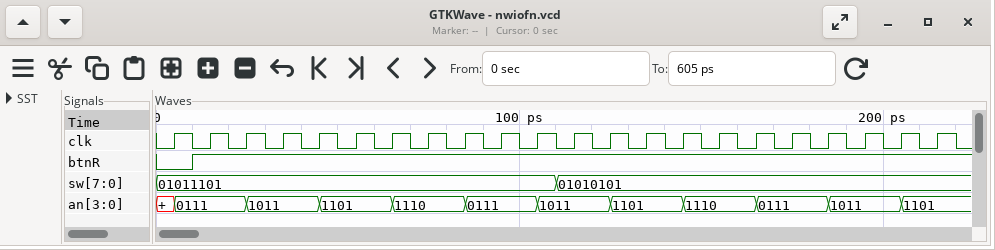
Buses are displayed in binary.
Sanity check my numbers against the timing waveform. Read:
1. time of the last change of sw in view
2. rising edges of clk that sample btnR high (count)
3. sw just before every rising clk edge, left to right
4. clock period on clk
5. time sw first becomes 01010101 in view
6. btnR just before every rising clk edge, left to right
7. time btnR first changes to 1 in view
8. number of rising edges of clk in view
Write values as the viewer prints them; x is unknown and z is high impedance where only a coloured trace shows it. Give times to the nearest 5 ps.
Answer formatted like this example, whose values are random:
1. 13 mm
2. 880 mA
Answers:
1. 110 ps
2. 21
3. 01011101, 01011101, 01011101, 01011101, 01011101, 01011101, 01011101, 01011101, 01011101, 01011101, 01011101, 01010101, 01010101, 01010101, 01010101, 01010101, 01010101, 01010101, 01010101, 01010101, 01010101, 01010101
4. 10 ps
5. 110 ps
6. 0 1 1 1 1 1 1 1 1 1 1 1 1 1 1 1 1 1 1 1 1 1
7. 10 ps
8. 22
